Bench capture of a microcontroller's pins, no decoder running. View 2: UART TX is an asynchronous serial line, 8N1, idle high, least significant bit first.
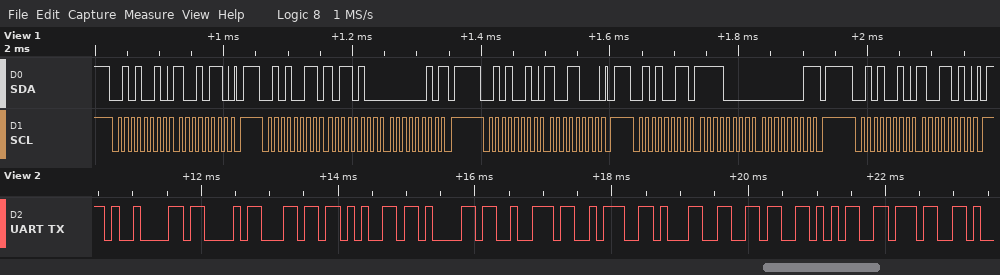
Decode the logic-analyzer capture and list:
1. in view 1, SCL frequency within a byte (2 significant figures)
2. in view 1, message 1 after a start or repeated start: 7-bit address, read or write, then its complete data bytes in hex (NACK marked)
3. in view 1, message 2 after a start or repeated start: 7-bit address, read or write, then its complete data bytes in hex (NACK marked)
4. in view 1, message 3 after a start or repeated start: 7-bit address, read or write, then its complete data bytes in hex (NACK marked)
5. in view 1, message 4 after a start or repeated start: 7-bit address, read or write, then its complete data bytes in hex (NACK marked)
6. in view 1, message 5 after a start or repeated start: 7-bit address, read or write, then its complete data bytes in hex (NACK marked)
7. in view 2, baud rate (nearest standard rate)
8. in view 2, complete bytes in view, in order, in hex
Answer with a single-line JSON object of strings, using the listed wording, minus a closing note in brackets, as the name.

{"in view 1, SCL frequency within a byte": "100 kHz", "in view 1, message 1 after a start or repeated start: 7-bit address, read or write, then its complete data bytes in hex": "0x29 write: 96", "in view 1, message 2 after a start or repeated start: 7-bit address, read or write, then its complete data bytes in hex": "0x29 read: B4 02 NACK", "in view 1, message 3 after a start or repeated start: 7-bit address, read or write, then its complete data bytes in hex": "0x29 write: 98", "in view 1, message 4 after a start or repeated start: 7-bit address, read or write, then its complete data bytes in hex": "0x29 read: F0 01 NACK", "in view 1, message 5 after a start or repeated start: 7-bit address, read or write, then its complete data bytes in hex": "0x29 write: 9A", "in view 2, baud rate": "9600 baud", "in view 2, complete bytes in view, in order, in hex": "0x09 0x43 0x6C 0x65 0x61 0x72 0x3A 0x31 0x36 0x35 0x37"}
